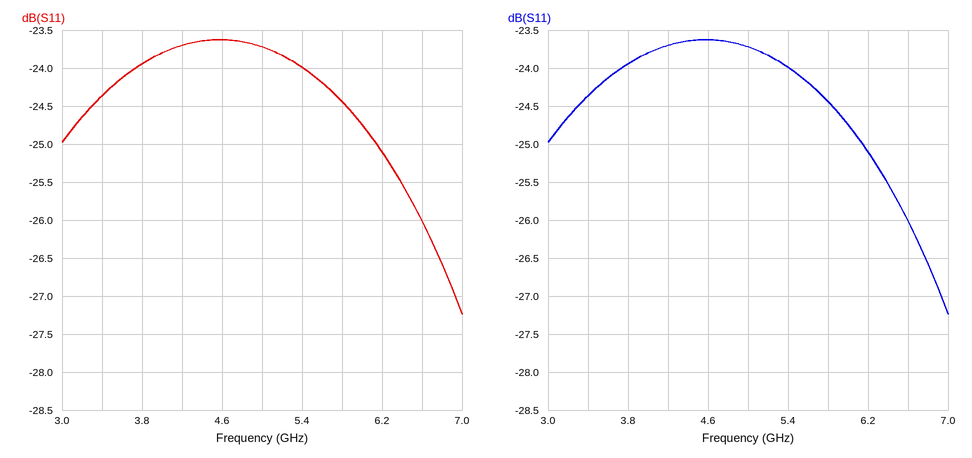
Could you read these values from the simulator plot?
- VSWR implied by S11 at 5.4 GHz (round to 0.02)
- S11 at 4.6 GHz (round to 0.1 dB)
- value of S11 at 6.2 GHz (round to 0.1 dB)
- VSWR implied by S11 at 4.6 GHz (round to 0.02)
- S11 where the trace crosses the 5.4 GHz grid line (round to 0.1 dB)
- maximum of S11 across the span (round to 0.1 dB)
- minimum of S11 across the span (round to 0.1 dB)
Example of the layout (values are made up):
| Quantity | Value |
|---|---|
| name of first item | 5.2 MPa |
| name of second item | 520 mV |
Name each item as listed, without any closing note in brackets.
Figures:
| Quantity | Value |
|---|---|
| VSWR implied by S11 at 5.4 GHz | 1.14 |
| S11 at 4.6 GHz | -23.6 dB |
| value of S11 at 6.2 GHz | -25.1 dB |
| VSWR implied by S11 at 4.6 GHz | 1.14 |
| S11 where the trace crosses the 5.4 GHz grid line | -24.0 dB |
| maximum of S11 across the span | -23.6 dB |
| minimum of S11 across the span | -27.2 dB |
